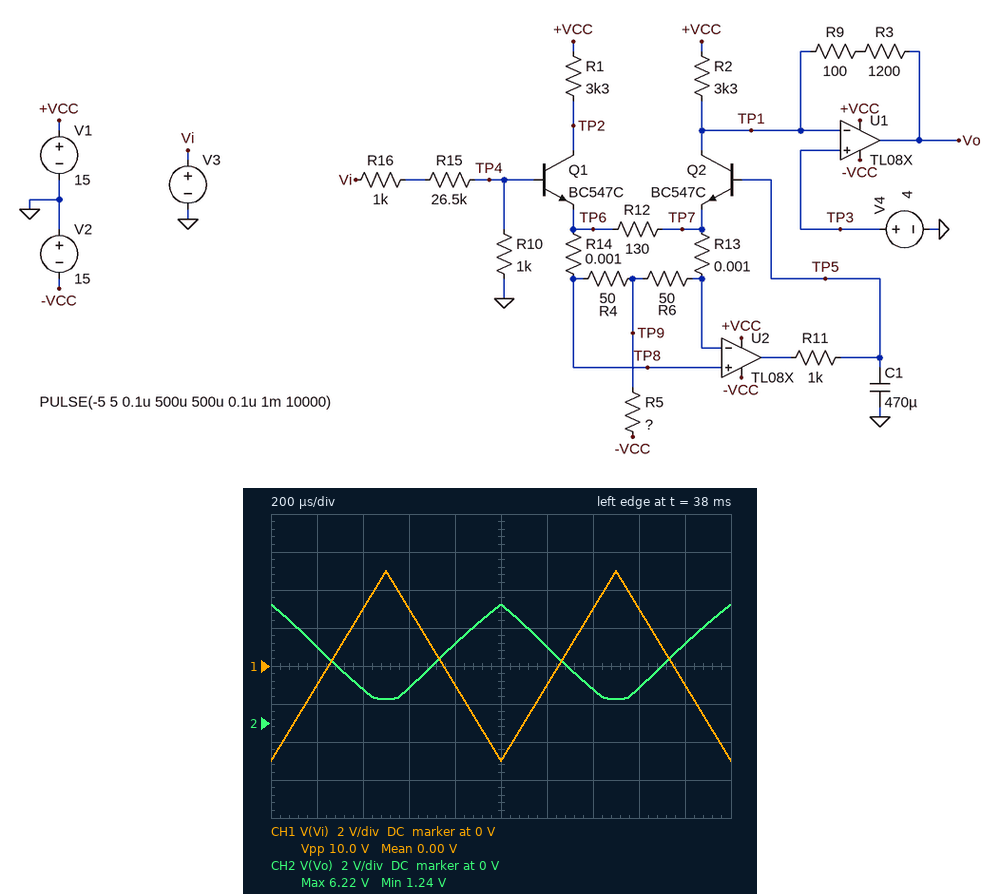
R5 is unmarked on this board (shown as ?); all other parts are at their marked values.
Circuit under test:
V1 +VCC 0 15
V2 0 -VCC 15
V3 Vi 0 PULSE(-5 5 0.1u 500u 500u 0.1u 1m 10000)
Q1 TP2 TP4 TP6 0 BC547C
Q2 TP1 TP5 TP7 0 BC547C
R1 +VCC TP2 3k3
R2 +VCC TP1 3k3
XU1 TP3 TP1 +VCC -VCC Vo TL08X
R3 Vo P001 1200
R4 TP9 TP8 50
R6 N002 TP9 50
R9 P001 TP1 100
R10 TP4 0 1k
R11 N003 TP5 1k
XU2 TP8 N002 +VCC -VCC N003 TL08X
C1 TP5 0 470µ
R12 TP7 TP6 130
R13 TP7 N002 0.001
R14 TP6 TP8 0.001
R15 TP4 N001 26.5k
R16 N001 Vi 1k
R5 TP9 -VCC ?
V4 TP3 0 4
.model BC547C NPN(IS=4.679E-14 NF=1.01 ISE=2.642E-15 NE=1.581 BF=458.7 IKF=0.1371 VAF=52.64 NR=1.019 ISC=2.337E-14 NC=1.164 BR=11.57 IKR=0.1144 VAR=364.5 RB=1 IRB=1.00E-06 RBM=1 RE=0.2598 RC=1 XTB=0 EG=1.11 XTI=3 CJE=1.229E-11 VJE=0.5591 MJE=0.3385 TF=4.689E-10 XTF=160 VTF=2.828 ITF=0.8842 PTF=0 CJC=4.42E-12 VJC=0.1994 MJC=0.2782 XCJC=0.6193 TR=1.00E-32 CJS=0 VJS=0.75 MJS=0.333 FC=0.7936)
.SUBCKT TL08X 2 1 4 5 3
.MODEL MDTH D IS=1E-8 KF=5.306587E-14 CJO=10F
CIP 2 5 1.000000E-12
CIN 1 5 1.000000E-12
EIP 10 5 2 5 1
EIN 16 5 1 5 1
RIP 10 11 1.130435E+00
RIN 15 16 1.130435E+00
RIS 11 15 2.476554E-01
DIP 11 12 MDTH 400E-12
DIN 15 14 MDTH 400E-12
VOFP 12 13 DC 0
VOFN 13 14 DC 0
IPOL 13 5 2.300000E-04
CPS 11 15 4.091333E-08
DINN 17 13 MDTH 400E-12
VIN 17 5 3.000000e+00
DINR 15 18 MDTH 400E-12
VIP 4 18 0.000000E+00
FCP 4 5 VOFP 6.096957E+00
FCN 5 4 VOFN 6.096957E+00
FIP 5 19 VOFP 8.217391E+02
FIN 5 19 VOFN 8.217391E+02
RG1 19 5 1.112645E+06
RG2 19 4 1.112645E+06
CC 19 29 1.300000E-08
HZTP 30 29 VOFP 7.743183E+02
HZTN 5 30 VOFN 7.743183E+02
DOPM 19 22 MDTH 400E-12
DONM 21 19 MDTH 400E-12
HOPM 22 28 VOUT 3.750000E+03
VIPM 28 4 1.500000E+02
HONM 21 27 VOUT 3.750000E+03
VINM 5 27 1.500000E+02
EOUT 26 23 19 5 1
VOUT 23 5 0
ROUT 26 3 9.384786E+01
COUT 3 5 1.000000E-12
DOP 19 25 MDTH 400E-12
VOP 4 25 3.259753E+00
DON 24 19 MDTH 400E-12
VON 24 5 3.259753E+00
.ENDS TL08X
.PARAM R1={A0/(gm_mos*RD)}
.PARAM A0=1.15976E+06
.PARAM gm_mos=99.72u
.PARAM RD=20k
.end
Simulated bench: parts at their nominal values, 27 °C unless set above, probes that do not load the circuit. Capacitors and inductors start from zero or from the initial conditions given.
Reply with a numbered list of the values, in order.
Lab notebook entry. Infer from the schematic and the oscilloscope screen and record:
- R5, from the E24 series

1. 2.4 kΩ
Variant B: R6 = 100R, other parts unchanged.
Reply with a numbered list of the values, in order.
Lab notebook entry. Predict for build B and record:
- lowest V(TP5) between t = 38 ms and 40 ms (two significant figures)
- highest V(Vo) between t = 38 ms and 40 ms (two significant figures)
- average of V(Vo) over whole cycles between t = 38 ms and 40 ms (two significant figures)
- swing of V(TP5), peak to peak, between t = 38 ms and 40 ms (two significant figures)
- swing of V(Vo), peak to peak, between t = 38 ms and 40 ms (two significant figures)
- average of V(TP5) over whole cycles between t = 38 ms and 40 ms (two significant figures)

1. -34 mV
2. 4.7 V
3. 2.4 V
4. 12 mV
5. 3.6 V
6. -28 mV
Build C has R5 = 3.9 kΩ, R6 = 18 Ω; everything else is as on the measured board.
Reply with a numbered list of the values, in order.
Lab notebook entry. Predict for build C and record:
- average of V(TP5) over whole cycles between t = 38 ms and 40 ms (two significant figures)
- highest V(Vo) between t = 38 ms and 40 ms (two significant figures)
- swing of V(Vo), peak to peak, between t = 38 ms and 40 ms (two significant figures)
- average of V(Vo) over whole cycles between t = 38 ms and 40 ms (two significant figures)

1. 29 mV
2. 4.4 V
3. 4.0 V
4. 2.9 V
